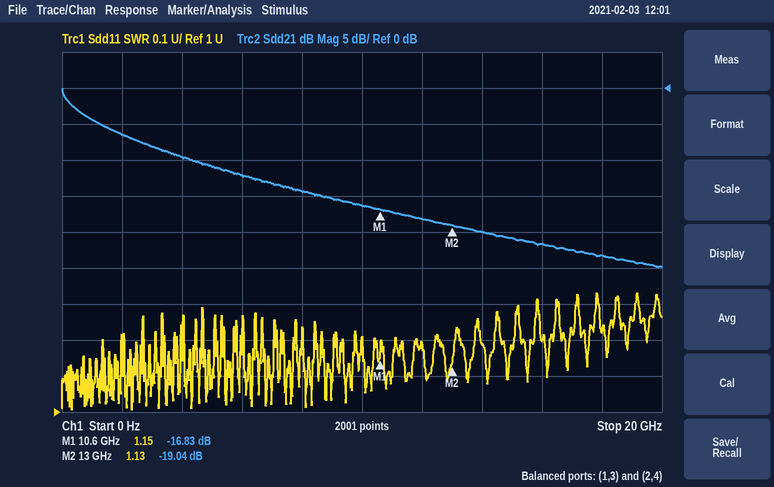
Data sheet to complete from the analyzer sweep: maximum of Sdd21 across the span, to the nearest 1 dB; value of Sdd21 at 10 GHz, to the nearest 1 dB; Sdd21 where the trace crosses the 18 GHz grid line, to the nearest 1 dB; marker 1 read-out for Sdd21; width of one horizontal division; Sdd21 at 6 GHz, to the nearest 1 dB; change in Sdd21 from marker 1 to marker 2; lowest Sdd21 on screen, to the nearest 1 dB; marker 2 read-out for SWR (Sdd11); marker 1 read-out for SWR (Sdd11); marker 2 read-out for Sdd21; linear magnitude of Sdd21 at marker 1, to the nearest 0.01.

0 dB
-16 dB
-23 dB
-16.83 dB
2 GHz
-12 dB
-2.21 dB
-25 dB
1.13
1.15
-19.04 dB
0.14
